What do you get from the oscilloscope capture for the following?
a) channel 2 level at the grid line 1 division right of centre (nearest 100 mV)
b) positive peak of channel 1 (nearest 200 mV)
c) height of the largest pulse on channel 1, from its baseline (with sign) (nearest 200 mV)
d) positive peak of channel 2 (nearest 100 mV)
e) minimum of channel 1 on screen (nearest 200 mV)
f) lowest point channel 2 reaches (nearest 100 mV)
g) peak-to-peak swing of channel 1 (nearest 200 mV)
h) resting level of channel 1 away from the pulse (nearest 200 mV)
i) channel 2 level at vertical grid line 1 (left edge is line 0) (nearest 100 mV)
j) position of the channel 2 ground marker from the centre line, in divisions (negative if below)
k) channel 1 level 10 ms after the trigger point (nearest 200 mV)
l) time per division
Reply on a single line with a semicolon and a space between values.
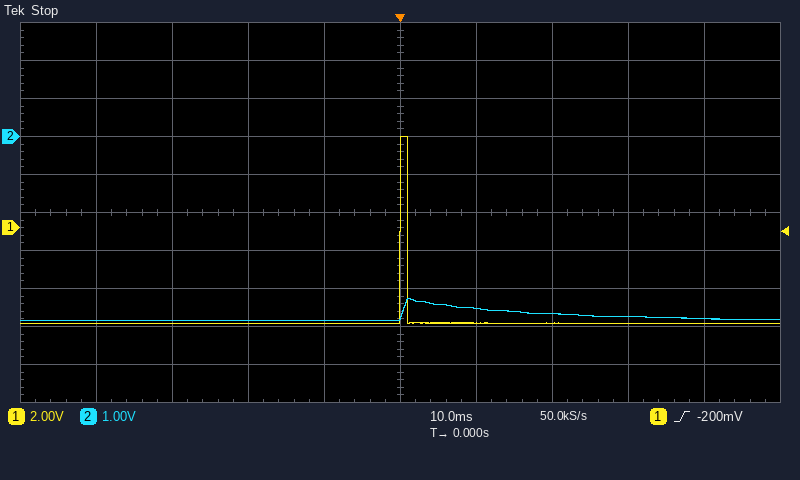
-4.5 V; 4.8 V; +9.8 V; -4.3 V; -5.0 V; -4.8 V; 9.8 V; -5.0 V; -4.8 V; +2.0 div; -5.0 V; 10 ms
